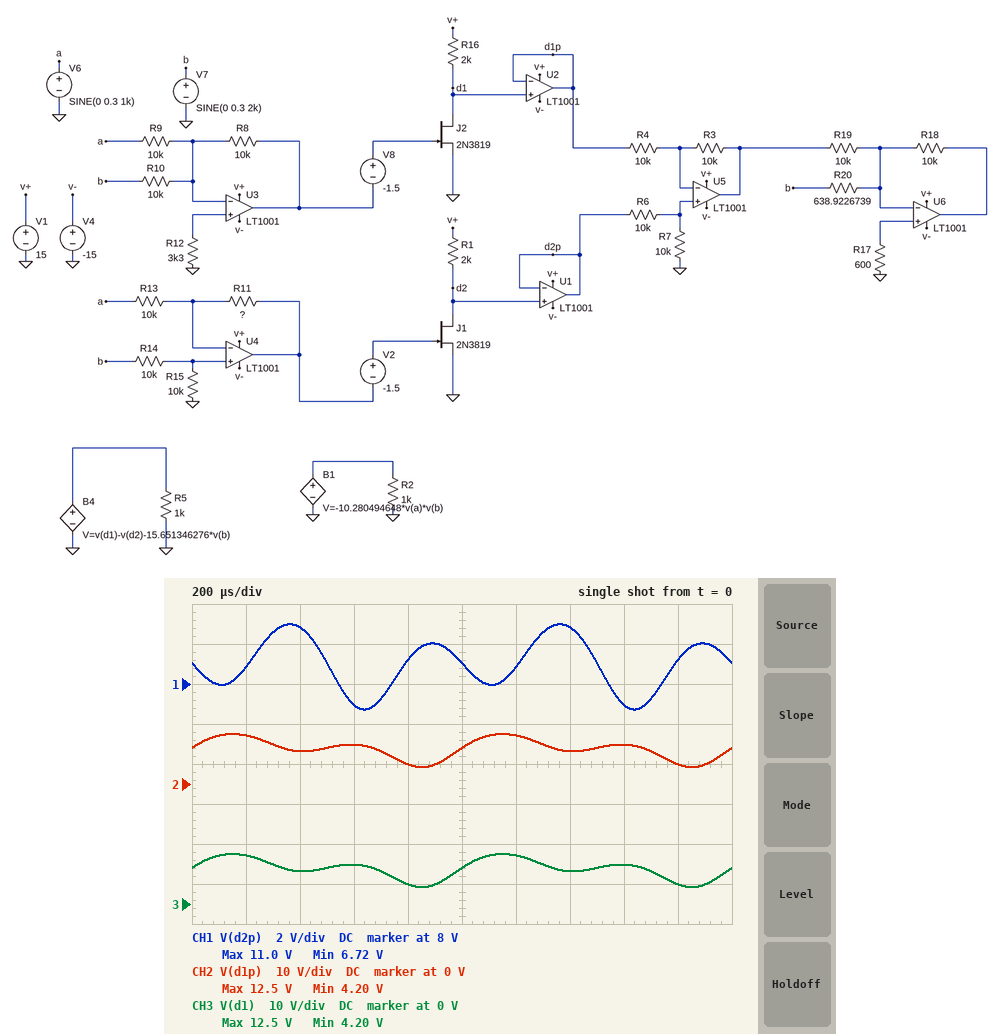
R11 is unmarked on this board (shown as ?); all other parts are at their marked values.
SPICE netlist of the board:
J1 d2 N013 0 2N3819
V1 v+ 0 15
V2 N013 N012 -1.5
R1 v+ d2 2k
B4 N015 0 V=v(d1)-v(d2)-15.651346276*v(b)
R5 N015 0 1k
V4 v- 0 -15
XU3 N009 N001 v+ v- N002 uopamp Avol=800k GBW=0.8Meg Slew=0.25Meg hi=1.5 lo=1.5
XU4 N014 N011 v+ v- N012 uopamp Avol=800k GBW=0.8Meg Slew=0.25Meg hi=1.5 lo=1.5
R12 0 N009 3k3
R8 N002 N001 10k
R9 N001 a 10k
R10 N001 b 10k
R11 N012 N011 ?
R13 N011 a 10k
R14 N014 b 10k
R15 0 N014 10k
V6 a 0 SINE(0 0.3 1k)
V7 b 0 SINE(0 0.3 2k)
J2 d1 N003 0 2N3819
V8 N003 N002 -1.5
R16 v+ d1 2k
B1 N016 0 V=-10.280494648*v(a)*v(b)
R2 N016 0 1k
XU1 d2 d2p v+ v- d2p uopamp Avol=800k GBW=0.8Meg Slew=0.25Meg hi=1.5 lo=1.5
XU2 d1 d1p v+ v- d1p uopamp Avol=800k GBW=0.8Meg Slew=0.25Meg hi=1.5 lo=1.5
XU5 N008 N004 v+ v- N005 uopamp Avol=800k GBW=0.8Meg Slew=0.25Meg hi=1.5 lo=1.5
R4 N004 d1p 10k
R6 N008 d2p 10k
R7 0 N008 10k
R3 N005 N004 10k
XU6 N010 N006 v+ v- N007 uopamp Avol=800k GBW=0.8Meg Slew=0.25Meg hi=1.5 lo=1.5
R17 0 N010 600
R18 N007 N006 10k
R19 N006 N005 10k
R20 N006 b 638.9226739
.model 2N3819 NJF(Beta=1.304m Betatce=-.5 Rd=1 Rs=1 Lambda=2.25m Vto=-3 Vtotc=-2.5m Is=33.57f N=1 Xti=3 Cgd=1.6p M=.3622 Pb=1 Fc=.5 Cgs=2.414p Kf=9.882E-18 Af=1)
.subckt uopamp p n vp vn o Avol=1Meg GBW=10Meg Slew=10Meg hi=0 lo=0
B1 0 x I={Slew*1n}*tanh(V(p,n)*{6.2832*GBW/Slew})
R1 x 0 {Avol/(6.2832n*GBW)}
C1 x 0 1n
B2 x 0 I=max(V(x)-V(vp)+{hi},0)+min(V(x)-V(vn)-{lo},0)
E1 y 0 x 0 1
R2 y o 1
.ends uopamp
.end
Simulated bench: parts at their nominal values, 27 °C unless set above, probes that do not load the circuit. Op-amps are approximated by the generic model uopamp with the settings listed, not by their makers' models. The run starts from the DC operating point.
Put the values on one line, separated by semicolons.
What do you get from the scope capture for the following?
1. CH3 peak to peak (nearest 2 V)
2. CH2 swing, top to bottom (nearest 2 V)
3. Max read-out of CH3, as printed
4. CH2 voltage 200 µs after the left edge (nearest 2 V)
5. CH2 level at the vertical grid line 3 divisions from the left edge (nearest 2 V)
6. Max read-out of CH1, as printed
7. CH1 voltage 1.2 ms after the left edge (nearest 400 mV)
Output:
8 V; 8 V; 12.5 V; 12 V; 10 V; 11.0 V; 8.8 V
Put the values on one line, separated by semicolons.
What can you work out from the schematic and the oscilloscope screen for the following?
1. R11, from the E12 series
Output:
3.3 kΩ
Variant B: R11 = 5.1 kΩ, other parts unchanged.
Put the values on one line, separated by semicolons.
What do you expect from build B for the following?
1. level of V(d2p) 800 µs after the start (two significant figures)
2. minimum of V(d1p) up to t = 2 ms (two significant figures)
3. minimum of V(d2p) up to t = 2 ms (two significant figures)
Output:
8.9 V; 4.2 V; 6.1 V
